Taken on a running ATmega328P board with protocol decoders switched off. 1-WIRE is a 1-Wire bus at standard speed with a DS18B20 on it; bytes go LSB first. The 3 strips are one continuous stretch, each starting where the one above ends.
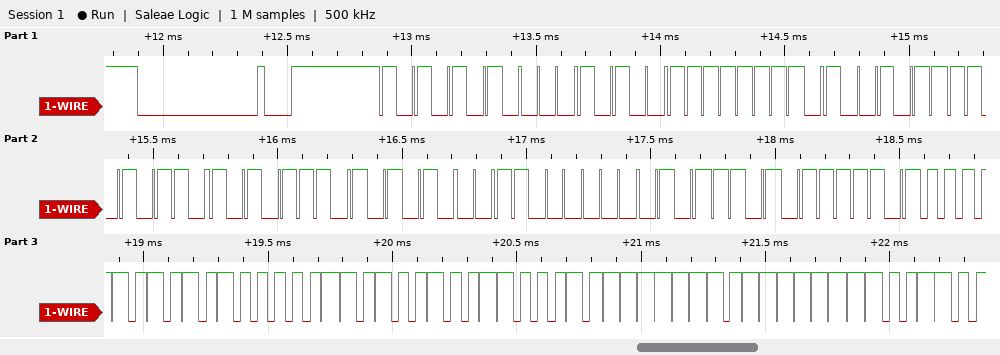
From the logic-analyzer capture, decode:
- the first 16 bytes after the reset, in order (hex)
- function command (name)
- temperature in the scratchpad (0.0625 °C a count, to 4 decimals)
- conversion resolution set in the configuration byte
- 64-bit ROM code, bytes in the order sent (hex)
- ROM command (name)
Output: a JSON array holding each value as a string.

["55 28 FF D2 6B 75 15 03 BA BE 50 05 4B 46 7F FF", "Read Scratchpad", "85.0000 °C", "12 bits", "28 FF D2 6B 75 15 03 BA", "Match ROM"]
